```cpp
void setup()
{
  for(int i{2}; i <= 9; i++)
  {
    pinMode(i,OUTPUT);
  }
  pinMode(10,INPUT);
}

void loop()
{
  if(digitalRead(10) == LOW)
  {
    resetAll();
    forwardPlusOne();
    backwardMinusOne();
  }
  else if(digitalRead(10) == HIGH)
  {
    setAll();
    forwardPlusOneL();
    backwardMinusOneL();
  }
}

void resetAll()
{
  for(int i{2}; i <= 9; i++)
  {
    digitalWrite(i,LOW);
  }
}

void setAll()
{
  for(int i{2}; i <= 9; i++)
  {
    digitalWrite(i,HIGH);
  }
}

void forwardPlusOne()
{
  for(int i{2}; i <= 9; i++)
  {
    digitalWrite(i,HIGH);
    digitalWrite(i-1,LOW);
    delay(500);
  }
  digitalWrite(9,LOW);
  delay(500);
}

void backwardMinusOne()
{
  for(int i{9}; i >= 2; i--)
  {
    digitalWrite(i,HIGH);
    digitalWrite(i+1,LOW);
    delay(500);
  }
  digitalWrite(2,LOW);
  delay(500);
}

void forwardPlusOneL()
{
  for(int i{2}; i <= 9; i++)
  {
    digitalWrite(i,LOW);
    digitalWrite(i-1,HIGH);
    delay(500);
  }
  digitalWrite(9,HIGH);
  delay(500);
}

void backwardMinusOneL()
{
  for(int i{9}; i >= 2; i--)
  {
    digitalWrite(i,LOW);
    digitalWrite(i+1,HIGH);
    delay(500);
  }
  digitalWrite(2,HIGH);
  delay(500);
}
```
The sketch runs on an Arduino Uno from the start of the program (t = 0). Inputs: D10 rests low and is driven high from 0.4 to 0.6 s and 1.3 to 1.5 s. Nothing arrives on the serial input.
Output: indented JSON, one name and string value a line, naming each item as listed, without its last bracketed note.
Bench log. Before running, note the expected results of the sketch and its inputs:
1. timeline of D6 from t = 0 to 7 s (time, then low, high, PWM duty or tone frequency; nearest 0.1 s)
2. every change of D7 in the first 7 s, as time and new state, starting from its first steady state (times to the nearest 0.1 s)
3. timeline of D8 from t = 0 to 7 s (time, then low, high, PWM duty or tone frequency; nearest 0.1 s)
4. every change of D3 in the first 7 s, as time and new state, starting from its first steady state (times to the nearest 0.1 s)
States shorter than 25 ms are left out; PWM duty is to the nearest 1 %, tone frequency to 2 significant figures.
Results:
{
  "timeline of D6 from t = 0 to 7 s": "0 s low; 2 s high; 2.5 s low; 6 s high; 6.5 s low",
  "every change of D7 in the first 7 s, as time and new state, starting from its first steady state": "0 s low; 2.5 s high; 3 s low; 5.5 s high; 6 s low",
  "timeline of D8 from t = 0 to 7 s": "0 s low; 3 s high; 3.5 s low; 5 s high; 5.5 s low",
  "every change of D3 in the first 7 s, as time and new state, starting from its first steady state": "0 s low; 0.5 s high; 1 s low"
}
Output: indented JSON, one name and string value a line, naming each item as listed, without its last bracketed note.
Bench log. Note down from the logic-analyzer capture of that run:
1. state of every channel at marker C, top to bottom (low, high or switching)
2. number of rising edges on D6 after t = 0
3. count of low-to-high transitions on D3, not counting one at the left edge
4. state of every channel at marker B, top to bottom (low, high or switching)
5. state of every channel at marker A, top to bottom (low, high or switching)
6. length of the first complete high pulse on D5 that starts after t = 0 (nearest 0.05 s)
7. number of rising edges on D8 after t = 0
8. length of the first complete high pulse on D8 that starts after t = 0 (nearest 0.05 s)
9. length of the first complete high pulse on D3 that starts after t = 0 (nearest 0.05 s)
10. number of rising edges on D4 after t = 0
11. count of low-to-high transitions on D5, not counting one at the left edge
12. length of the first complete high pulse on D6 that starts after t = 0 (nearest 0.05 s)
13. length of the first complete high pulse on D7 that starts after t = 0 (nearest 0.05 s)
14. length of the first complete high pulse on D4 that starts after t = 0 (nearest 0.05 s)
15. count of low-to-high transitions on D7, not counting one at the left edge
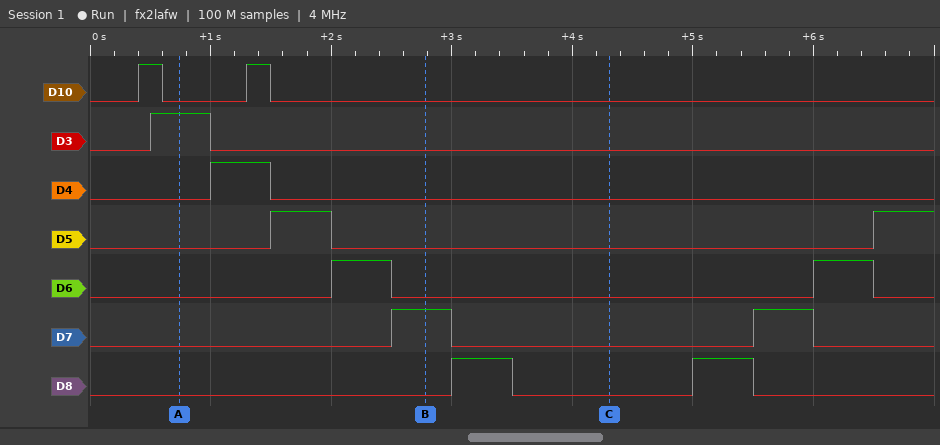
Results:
{
  "state of every channel at marker C, top to bottom": "D10 low, D3 low, D4 low, D5 low, D6 low, D7 low, D8 low",
  "number of rising edges on D6 after t = 0": "2",
  "count of low-to-high transitions on D3, not counting one at the left edge": "1",
  "state of every channel at marker B, top to bottom": "D10 low, D3 low, D4 low, D5 low, D6 low, D7 high, D8 low",
  "state of every channel at marker A, top to bottom": "D10 low, D3 high, D4 low, D5 low, D6 low, D7 low, D8 low",
  "length of the first complete high pulse on D5 that starts after t = 0": "0.50 s",
  "number of rising edges on D8 after t = 0": "2",
  "length of the first complete high pulse on D8 that starts after t = 0": "0.50 s",
  "length of the first complete high pulse on D3 that starts after t = 0": "0.50 s",
  "number of rising edges on D4 after t = 0": "1",
  "count of low-to-high transitions on D5, not counting one at the left edge": "2",
  "length of the first complete high pulse on D6 that starts after t = 0": "0.50 s",
  "length of the first complete high pulse on D7 that starts after t = 0": "0.50 s",
  "length of the first complete high pulse on D4 that starts after t = 0": "0.50 s",
  "count of low-to-high transitions on D7, not counting one at the left edge": "2"
}
